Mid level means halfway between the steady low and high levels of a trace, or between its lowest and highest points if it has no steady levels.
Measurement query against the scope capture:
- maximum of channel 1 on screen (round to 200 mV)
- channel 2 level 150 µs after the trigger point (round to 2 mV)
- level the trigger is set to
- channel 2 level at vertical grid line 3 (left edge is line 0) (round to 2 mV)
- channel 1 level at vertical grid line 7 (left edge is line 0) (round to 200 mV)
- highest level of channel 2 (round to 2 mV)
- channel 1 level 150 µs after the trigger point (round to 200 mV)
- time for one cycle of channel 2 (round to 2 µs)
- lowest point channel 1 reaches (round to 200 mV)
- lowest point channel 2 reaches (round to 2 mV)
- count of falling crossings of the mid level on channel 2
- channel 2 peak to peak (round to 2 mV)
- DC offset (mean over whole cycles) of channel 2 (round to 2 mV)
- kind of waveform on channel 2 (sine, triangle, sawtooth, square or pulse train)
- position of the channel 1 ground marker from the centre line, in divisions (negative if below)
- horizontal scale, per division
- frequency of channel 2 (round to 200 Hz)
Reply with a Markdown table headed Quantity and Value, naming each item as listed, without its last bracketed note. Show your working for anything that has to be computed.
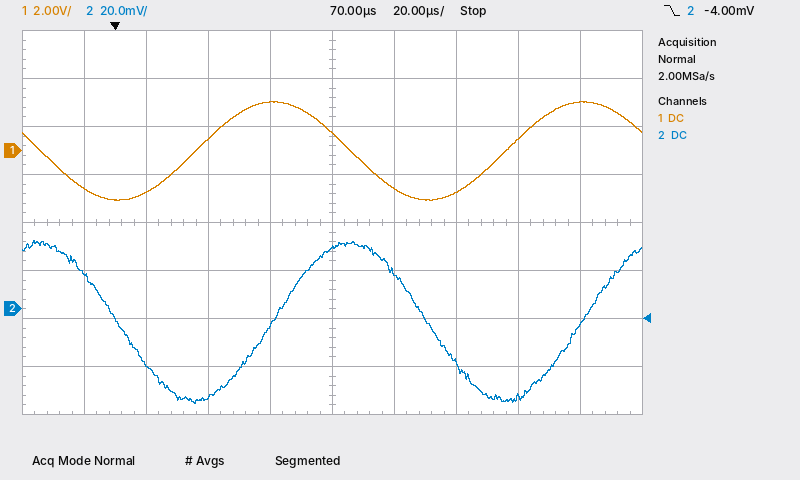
| Quantity | Value |
|---|---|
| maximum of channel 1 on screen | 2.0 V |
| channel 2 level 150 µs after the trigger point | -6 mV |
| level the trigger is set to | -4.00 mV |
| channel 2 level at vertical grid line 3 (left edge is line 0) | -36 mV |
| channel 1 level at vertical grid line 7 (left edge is line 0) | -1.8 V |
| highest level of channel 2 | 28 mV |
| channel 1 level 150 µs after the trigger point | 2.0 V |
| time for one cycle of channel 2 | 100 µs |
| lowest point channel 1 reaches | -2.0 V |
| lowest point channel 2 reaches | -40 mV |
| count of falling crossings of the mid level on channel 2 | 2 |
| channel 2 peak to peak | 28 mV − (-40 mV) = 68 mV |
| DC offset (mean over whole cycles) of channel 2 | (28 mV + (-40 mV)) / 2 ≈ -6 mV |
| kind of waveform on channel 2 | sine |
| position of the channel 1 ground marker from the centre line, in divisions | +1.5 div |
| horizontal scale, per division | 20 µs |
| frequency of channel 2 | 1 / 100 µs ≈ 10.0 kHz |
